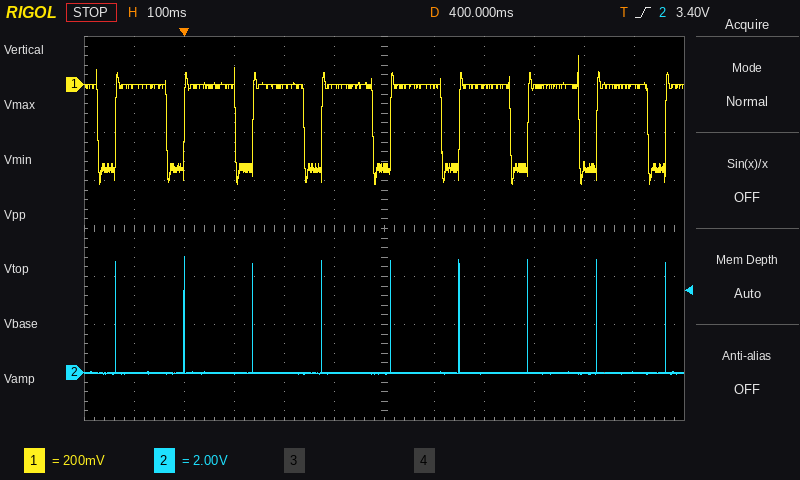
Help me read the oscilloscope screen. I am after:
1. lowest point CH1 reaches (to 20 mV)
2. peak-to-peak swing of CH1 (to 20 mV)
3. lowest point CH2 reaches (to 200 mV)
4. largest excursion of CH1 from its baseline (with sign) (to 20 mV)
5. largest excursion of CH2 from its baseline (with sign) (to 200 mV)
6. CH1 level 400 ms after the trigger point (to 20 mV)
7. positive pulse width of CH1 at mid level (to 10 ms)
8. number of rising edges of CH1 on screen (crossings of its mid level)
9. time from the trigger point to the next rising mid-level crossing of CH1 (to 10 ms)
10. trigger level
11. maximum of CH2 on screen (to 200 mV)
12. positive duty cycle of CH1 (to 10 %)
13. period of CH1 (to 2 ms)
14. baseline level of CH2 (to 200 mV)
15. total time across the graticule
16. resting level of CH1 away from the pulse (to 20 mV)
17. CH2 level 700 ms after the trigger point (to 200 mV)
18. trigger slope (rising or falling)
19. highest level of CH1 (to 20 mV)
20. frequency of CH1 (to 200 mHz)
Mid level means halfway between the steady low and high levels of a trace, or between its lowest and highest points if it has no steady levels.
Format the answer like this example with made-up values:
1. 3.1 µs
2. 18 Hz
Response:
1. -420 mV
2. 540 mV
3. 0.0 V
4. -420 mV
5. +4.8 V
6. -340 mV
7. 100 ms
8. 9
9. 140 ms
10. 3.40 V
11. 4.8 V
12. 70 %
13. 138 ms
14. 0.0 V
15. 1.2 s
16. 0 mV
17. 0.0 V
18. rising
19. 120 mV
20. 7.2 Hz
